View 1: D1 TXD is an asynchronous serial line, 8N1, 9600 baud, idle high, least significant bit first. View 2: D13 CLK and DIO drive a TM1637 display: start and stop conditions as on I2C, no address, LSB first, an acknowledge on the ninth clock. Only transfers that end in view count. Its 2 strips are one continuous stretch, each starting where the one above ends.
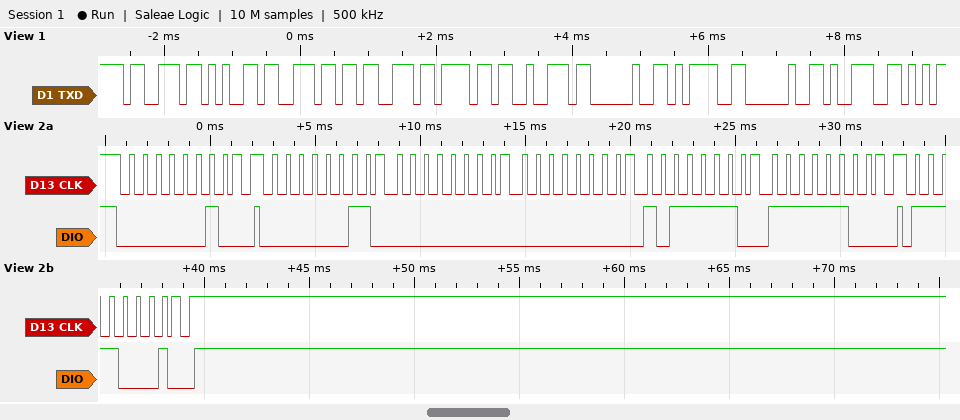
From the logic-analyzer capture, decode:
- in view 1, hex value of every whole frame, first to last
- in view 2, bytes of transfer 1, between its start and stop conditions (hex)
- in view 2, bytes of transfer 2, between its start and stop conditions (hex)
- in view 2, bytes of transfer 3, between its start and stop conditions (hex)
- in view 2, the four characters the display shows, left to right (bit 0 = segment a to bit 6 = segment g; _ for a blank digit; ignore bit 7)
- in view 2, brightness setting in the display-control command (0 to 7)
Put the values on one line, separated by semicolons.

73 65 6E 73 6F 72 20 3D 20 39; 40; C0 00 00 7D 3F; 8F; __60; 7
